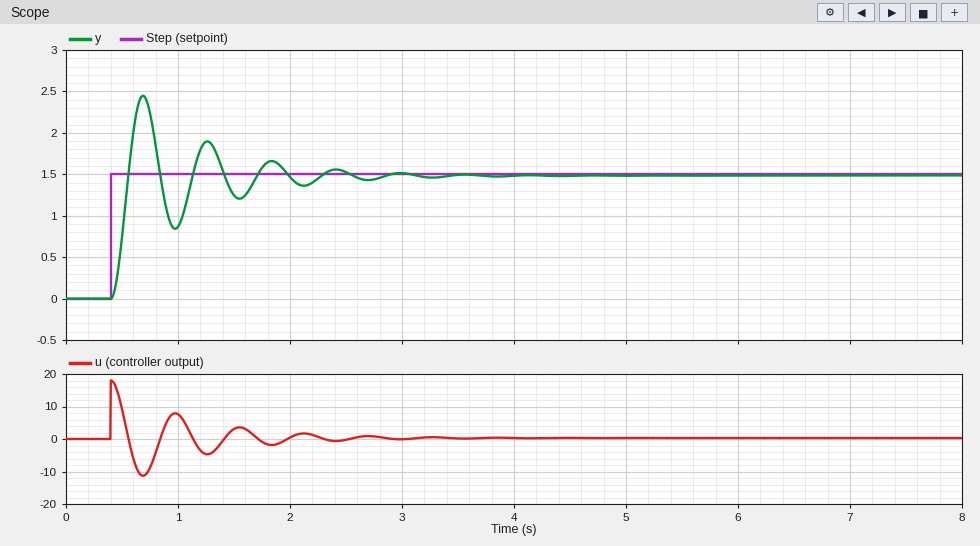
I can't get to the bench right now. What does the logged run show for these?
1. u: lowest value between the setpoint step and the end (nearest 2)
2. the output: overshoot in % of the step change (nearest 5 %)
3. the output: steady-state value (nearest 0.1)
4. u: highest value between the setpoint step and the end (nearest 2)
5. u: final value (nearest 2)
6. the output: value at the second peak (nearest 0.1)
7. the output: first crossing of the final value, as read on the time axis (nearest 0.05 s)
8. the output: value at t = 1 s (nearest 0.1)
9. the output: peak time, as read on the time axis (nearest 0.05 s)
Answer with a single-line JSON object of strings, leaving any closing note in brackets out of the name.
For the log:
{"u: lowest value between the setpoint step and the end": "-12", "the output: overshoot in % of the step change": "65 %", "the output: steady-state value": "1.5", "u: highest value between the setpoint step and the end": "18", "u: final value": "0", "the output: value at the second peak": "1.9", "the output: first crossing of the final value, as read on the time axis": "0.55 s", "the output: value at t = 1 s": "0.9", "the output: peak time, as read on the time axis": "0.70 s"}
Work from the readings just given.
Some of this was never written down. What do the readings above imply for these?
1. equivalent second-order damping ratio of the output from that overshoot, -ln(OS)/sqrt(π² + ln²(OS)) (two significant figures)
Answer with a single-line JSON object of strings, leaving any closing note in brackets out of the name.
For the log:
{"equivalent second-order damping ratio of the output from that overshoot, -ln(OS)/sqrt(π² + ln²(OS))": "0.14"}
